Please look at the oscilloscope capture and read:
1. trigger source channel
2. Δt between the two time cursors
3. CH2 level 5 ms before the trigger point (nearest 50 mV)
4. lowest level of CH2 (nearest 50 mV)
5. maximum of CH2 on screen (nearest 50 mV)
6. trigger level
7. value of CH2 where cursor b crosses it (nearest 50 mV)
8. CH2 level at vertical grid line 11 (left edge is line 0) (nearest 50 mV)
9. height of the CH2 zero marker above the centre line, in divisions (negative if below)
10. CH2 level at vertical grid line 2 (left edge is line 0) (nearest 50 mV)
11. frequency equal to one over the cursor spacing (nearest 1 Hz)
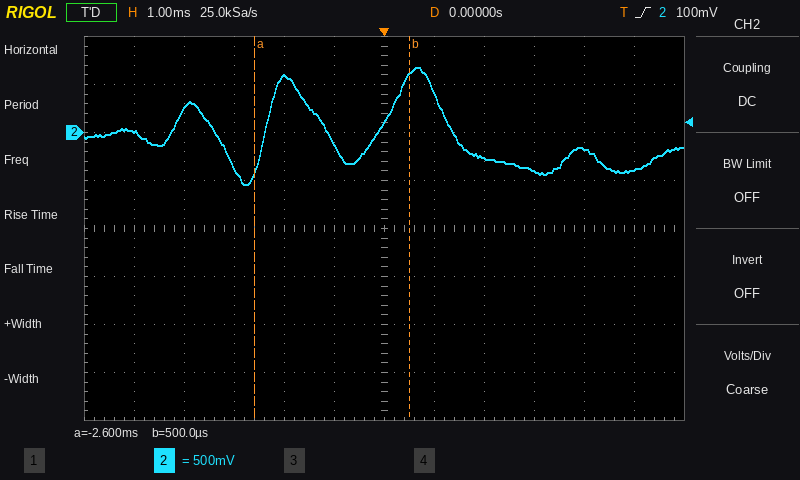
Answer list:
CH2
3.1 ms
0 mV
-550 mV
700 mV
100 mV
600 mV
-400 mV
+2.0 div
250 mV
323 Hz
